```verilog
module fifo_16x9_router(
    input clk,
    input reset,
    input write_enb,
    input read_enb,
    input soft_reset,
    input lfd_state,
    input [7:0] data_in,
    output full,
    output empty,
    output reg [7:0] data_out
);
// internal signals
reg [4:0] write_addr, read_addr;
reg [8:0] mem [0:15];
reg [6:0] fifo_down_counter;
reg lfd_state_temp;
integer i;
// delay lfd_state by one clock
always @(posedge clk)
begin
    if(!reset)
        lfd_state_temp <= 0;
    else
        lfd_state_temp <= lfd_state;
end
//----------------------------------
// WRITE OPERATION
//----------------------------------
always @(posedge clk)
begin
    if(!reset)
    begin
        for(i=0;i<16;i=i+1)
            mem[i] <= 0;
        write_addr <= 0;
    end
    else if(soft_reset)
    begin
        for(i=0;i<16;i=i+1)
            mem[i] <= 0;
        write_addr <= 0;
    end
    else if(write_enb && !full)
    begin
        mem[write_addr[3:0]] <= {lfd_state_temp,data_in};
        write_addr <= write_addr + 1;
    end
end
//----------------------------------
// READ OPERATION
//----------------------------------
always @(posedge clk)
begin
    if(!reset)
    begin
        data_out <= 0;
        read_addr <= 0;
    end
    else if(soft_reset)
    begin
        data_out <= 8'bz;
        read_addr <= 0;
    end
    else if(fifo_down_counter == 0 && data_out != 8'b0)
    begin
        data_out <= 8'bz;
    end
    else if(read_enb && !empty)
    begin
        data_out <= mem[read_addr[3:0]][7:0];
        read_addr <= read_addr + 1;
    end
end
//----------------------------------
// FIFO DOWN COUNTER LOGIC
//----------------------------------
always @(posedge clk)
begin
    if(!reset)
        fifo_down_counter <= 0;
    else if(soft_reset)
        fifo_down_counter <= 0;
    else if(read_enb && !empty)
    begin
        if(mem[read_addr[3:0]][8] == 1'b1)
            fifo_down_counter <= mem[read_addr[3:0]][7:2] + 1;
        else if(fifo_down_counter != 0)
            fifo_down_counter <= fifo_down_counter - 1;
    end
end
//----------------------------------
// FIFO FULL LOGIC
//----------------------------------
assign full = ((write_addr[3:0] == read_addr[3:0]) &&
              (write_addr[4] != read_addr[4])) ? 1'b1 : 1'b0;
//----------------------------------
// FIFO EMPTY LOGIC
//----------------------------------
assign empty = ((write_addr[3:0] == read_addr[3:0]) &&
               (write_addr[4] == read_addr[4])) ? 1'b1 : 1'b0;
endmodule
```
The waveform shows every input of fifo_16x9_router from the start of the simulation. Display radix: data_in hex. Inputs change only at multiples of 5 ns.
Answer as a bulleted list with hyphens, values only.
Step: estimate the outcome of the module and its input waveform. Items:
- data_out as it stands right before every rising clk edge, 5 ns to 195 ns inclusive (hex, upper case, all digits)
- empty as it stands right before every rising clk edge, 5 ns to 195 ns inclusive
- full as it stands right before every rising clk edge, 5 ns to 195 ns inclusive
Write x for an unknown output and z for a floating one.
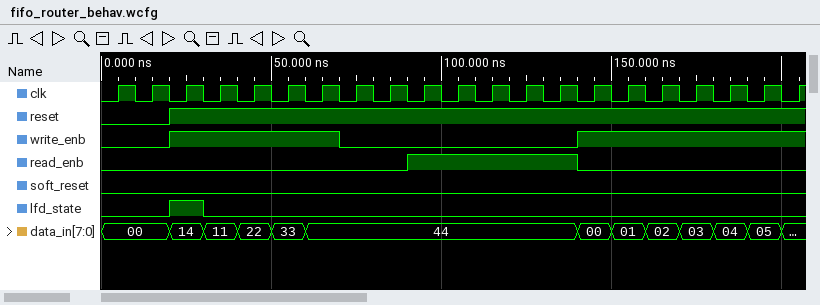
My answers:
- x, 00, 00, 00, 00, 00, 00, 00, 00, 00, 14, z, 11, 22, 33, 33, 33, 33, 33, 33
- x 1 1 0 0 0 0 0 0 0 0 0 0 0 0 0 0 0 0 0
- x 0 0 0 0 0 0 0 0 0 0 0 0 0 0 0 0 0 0 0
